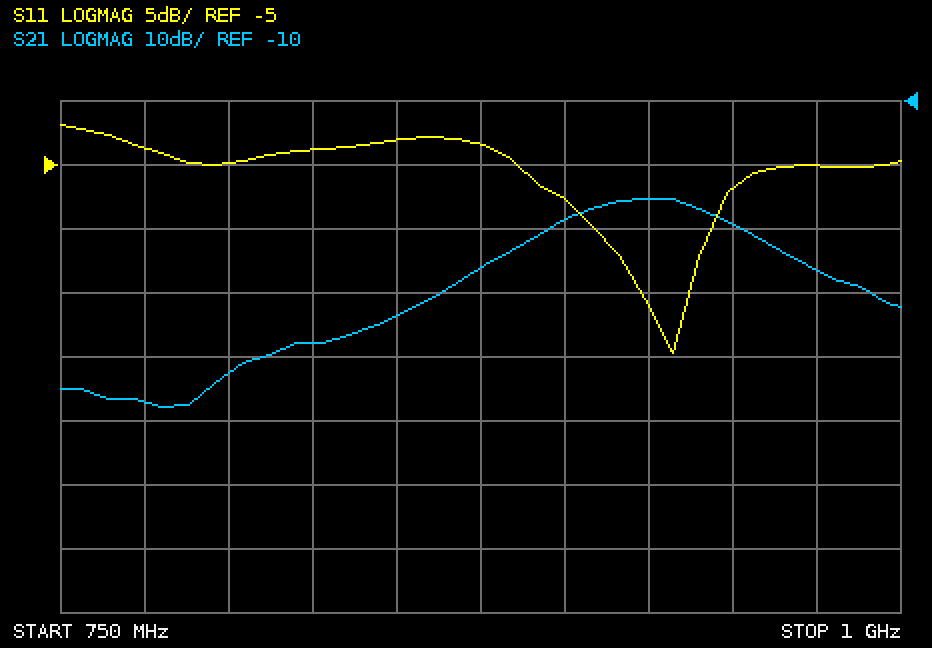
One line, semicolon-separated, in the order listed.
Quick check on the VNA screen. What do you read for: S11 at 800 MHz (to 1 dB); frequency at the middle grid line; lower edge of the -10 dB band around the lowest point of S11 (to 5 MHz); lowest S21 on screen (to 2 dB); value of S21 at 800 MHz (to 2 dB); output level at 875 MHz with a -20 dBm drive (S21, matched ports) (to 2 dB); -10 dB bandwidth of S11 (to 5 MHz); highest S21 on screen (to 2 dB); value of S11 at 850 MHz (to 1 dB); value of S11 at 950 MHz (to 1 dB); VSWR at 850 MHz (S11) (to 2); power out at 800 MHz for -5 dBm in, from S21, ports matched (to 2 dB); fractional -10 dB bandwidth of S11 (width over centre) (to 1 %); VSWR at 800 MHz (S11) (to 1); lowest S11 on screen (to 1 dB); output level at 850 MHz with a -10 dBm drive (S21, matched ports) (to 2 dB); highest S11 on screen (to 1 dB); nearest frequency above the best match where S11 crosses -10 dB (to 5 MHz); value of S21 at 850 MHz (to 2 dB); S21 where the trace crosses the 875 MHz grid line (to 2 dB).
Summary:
-5 dB; 875 MHz; 910 MHz; -58 dB; -52 dB; -56 dBm; 35 MHz; -26 dB; -3 dB; -7 dB; 6; -58 dBm; 4 %; 4; -20 dB; -54 dBm; -2 dB; 945 MHz; -44 dB; -36 dB
